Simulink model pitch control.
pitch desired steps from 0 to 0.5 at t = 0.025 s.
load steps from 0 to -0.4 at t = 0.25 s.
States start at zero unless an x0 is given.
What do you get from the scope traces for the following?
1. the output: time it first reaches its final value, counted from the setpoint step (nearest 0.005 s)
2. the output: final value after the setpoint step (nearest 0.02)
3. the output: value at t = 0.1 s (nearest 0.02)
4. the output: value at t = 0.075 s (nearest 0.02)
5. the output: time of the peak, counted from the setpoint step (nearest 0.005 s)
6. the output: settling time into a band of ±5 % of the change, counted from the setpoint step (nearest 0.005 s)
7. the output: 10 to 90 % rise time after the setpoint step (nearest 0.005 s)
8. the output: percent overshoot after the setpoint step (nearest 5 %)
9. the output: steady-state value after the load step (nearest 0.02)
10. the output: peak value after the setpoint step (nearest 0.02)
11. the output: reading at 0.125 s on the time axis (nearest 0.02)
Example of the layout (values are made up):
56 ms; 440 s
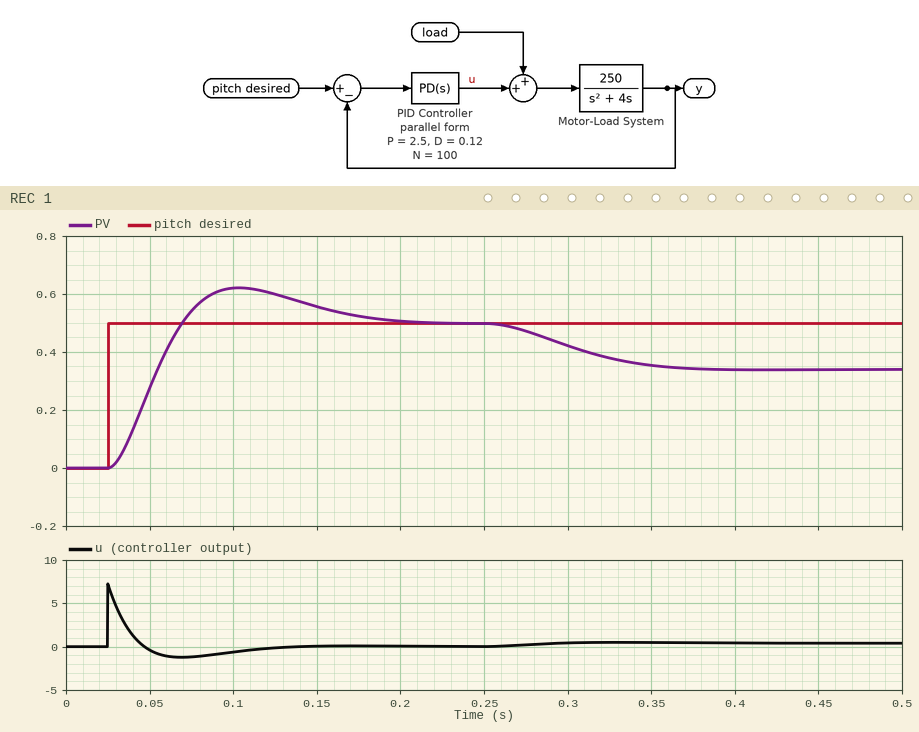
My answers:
0.045 s; 0.50; 0.62; 0.54; 0.080 s; 0.150 s; 0.030 s; 25 %; 0.34; 0.62; 0.60
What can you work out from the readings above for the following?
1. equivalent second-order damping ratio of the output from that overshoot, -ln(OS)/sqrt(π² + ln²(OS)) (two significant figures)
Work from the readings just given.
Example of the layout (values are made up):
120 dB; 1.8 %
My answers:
0.40
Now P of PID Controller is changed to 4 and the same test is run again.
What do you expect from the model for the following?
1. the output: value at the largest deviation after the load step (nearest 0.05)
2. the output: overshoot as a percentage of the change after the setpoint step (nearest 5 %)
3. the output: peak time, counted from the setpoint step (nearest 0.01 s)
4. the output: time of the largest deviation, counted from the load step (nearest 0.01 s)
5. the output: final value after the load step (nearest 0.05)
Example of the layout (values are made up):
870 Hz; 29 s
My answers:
0.40; 35 %; 0.07 s; 0.10 s; 0.40
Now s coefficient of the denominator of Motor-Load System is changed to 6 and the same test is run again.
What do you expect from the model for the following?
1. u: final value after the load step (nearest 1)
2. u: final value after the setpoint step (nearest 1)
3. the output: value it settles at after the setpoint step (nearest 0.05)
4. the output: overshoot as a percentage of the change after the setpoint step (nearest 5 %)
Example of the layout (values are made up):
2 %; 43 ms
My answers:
0; 0; 0.50; 20 %
